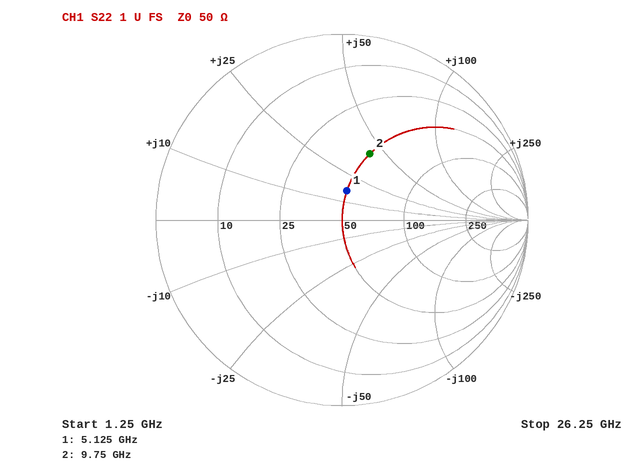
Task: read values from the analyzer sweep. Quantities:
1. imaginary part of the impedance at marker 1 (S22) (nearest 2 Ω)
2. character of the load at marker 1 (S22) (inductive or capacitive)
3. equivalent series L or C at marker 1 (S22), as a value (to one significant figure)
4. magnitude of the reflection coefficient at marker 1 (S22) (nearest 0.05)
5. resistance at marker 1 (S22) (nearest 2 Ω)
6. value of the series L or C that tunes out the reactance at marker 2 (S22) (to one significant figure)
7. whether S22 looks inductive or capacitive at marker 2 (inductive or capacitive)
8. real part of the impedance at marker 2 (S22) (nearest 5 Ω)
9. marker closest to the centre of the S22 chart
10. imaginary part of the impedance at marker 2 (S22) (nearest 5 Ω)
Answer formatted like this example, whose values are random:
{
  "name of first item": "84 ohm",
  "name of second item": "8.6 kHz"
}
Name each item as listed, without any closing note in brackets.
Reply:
{
  "imaginary part of the impedance at marker 1 (S22)": "+16 Ω",
  "character of the load at marker 1 (S22)": "inductive",
  "equivalent series L or C at marker 1 (S22), as a value": "500 pH",
  "magnitude of the reflection coefficient at marker 1 (S22)": "0.15",
  "resistance at marker 1 (S22)": "50 Ω",
  "value of the series L or C that tunes out the reactance at marker 2 (S22)": "400 fF",
  "whether S22 looks inductive or capacitive at marker 2": "inductive",
  "real part of the impedance at marker 2 (S22)": "50 Ω",
  "marker closest to the centre of the S22 chart": "marker 1",
  "imaginary part of the impedance at marker 2 (S22)": "+40 Ω"
}
